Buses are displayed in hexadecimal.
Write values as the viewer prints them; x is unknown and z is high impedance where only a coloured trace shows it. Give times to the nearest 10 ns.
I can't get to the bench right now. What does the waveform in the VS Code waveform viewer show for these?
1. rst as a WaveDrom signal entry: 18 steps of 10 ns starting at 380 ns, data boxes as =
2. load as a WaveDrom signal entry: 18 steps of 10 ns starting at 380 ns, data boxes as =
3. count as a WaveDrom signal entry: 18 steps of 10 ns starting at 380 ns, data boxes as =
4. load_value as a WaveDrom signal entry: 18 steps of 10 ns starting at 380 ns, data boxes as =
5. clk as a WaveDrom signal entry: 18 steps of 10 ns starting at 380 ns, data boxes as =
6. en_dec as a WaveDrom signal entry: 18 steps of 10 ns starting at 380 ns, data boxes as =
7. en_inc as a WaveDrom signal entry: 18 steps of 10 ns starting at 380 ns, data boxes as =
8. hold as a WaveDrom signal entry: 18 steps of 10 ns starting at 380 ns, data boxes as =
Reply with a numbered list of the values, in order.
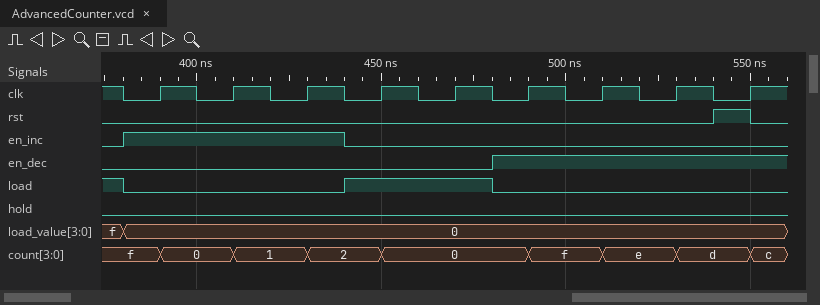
1. {name: 'rst', wave: '0...............10'}
2. {name: 'load', wave: '0.....1...0.......'}
3. {name: 'count', wave: '==.=.=.=...=.=.=.=', data: 'f 0 1 2 0 f e d c'}
4. {name: 'load_value', wave: '=.................', data: '0'}
5. {name: 'clk', wave: '010101010101010101'}
6. {name: 'en_dec', wave: '0.........1.......'}
7. {name: 'en_inc', wave: '1.....0...........'}
8. {name: 'hold', wave: '0.................'}
